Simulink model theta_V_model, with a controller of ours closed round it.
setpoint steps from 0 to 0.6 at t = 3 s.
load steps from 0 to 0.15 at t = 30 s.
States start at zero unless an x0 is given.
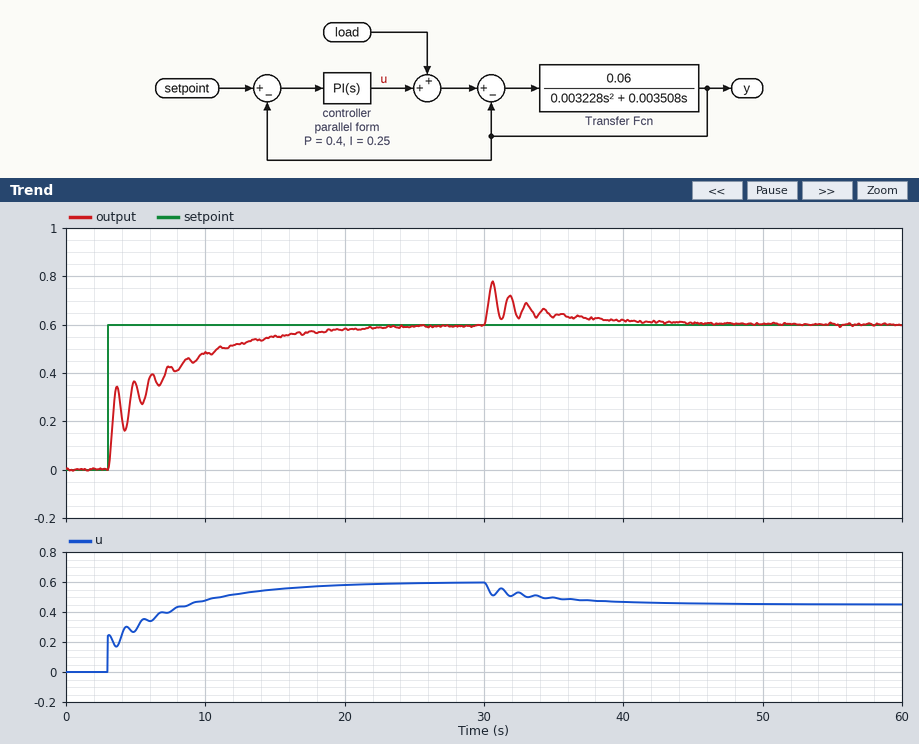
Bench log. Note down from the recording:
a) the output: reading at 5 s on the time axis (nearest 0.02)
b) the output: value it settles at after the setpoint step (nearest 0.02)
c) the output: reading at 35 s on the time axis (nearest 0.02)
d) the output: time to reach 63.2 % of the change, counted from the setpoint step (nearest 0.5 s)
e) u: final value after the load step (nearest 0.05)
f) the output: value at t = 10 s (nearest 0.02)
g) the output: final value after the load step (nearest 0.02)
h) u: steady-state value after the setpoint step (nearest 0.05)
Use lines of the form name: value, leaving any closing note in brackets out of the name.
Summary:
the output: reading at 5 s on the time axis: 0.36
the output: value it settles at after the setpoint step: 0.60
the output: reading at 35 s on the time axis: 0.64
the output: time to reach 63.2 % of the change, counted from the setpoint step: 3.0 s
u: final value after the load step: 0.45
the output: value at t = 10 s: 0.48
the output: final value after the load step: 0.60
u: steady-state value after the setpoint step: 0.60
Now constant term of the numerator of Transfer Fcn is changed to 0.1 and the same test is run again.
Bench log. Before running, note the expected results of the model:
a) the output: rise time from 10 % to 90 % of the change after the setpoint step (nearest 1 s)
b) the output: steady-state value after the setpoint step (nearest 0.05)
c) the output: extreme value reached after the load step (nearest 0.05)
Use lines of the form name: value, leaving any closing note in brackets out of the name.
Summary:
the output: rise time from 10 % to 90 % of the change after the setpoint step: 11 s
the output: steady-state value after the setpoint step: 0.60
the output: extreme value reached after the load step: 0.80
